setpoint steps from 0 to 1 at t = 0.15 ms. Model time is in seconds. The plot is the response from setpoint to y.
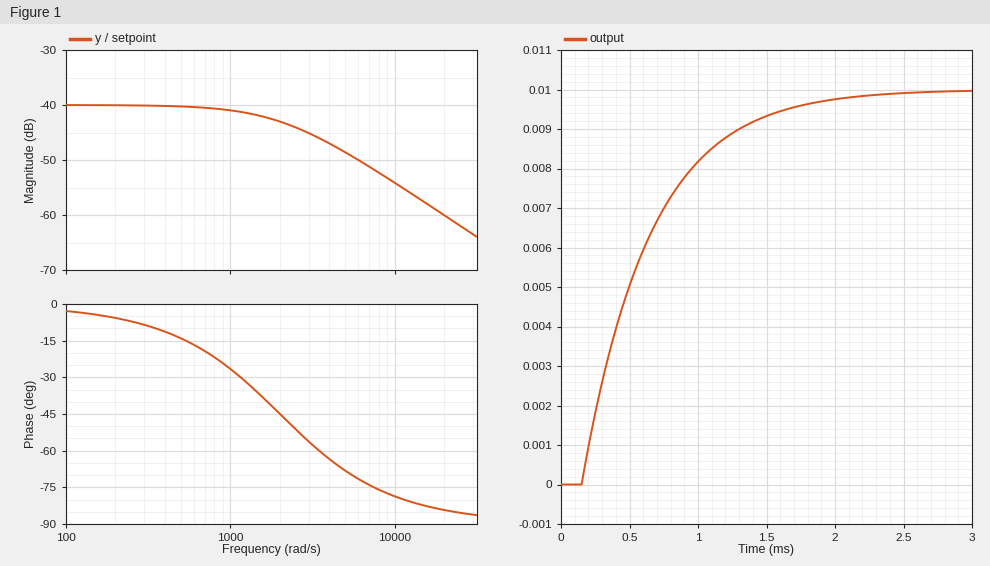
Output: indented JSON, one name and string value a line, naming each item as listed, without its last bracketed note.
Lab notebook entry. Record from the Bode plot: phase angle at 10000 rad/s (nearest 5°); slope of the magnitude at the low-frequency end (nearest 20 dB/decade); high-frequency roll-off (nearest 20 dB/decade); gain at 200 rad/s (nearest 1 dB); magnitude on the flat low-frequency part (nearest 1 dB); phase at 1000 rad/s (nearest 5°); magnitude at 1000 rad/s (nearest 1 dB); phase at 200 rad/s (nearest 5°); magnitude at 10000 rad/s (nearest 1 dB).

{
  "phase angle at 10000 rad/s": "-80°",
  "slope of the magnitude at the low-frequency end": "0 dB/decade",
  "high-frequency roll-off": "-20 dB/decade",
  "gain at 200 rad/s": "-40 dB",
  "magnitude on the flat low-frequency part": "-40 dB",
  "phase at 1000 rad/s": "-25°",
  "magnitude at 1000 rad/s": "-41 dB",
  "phase at 200 rad/s": "-5°",
  "magnitude at 10000 rad/s": "-54 dB"
}
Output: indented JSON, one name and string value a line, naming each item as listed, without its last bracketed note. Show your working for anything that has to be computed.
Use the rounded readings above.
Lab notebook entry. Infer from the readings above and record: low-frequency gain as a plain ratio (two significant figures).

{
  "low-frequency gain as a plain ratio": "10^(-40 / 20) = 0.010"
}
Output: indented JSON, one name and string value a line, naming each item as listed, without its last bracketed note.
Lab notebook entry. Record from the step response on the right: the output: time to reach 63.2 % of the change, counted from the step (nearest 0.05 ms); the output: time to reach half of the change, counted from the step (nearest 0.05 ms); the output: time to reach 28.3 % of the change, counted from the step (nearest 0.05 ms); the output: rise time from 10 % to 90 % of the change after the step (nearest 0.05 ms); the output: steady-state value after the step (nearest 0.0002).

{
  "the output: time to reach 63.2 % of the change, counted from the step": "0.50 ms",
  "the output: time to reach half of the change, counted from the step": "0.35 ms",
  "the output: time to reach 28.3 % of the change, counted from the step": "0.15 ms",
  "the output: rise time from 10 % to 90 % of the change after the step": "1.10 ms",
  "the output: steady-state value after the step": "0.0100"
}
